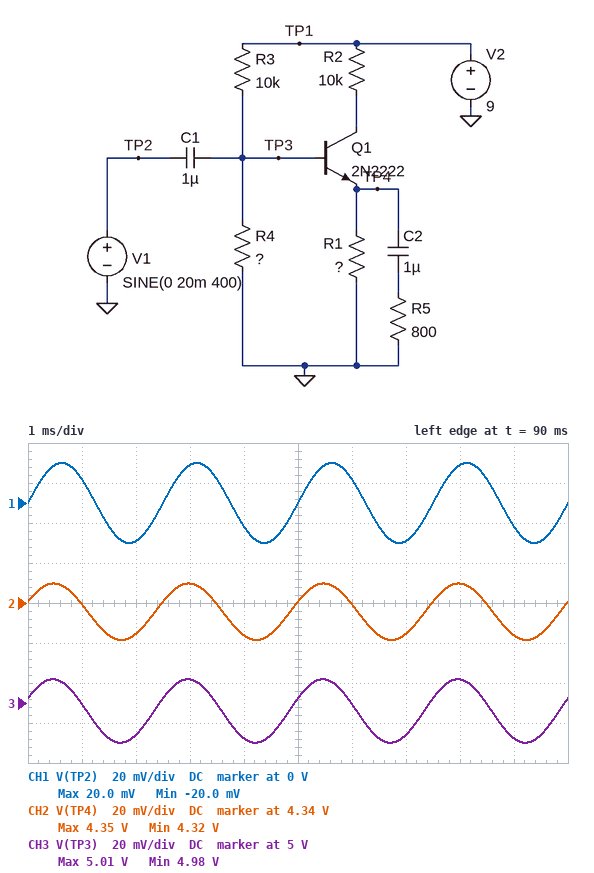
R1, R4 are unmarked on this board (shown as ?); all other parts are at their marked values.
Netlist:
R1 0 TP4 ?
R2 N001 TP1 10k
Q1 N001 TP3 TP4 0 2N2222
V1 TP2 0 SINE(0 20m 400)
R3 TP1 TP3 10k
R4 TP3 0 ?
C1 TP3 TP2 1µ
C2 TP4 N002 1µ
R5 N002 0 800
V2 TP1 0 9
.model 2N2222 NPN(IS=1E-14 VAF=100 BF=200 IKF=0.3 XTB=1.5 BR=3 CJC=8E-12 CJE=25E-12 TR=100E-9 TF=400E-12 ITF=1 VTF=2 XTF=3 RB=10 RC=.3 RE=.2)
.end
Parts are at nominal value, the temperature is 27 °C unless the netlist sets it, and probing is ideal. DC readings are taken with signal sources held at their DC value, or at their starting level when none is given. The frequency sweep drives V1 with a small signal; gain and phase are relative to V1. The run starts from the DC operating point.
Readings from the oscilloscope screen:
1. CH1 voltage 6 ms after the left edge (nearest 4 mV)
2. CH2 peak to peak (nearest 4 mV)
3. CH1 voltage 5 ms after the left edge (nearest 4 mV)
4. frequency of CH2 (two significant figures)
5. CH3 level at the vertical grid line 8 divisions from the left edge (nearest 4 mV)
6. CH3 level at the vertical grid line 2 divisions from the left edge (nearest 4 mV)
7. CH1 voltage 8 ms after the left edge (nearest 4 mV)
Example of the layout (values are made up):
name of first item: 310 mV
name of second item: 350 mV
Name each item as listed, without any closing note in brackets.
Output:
CH1 voltage 6 ms after the left edge: 12 mV
CH2 peak to peak: 28 mV
CH1 voltage 5 ms after the left edge: 0 V
frequency of CH2: 400 Hz
CH3 level at the vertical grid line 8 divisions from the left edge: 5.012 V
CH3 level at the vertical grid line 2 divisions from the left edge: 4.984 V
CH1 voltage 8 ms after the left edge: 20 mV
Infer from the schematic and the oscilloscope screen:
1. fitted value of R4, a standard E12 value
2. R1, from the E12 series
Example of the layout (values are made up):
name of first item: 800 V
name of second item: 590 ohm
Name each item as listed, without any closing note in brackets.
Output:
fitted value of R4, a standard E12 value: 22 kΩ
R1, from the E12 series: 6.8 kΩ
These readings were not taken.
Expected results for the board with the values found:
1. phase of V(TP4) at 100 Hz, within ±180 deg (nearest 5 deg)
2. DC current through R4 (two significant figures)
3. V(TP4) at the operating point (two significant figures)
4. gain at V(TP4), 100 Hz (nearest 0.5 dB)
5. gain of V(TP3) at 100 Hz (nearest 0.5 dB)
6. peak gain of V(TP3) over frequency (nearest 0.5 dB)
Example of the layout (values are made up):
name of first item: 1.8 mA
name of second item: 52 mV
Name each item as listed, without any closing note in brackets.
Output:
phase of V(TP4) at 100 Hz, within ±180 deg: 30 deg
DC current through R4: 230 µA
V(TP4) at the operating point: 4.3 V
gain at V(TP4), 100 Hz: -6.5 dB
gain of V(TP3) at 100 Hz: -6.0 dB
peak gain of V(TP3) over frequency: 0 dB
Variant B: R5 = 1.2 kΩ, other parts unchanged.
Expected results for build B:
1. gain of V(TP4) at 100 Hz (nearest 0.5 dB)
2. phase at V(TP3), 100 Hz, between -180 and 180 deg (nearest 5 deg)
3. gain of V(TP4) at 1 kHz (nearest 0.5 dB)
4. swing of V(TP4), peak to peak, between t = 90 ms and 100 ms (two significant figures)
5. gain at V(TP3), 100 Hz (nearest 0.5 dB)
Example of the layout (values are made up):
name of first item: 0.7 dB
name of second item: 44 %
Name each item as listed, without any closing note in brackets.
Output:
gain of V(TP4) at 100 Hz: -6.0 dB
phase at V(TP3), 100 Hz, between -180 and 180 deg: 35 deg
gain of V(TP4) at 1 kHz: -1.0 dB
swing of V(TP4), peak to peak, between t = 90 ms and 100 ms: 31 mV
gain at V(TP3), 100 Hz: -5.5 dB
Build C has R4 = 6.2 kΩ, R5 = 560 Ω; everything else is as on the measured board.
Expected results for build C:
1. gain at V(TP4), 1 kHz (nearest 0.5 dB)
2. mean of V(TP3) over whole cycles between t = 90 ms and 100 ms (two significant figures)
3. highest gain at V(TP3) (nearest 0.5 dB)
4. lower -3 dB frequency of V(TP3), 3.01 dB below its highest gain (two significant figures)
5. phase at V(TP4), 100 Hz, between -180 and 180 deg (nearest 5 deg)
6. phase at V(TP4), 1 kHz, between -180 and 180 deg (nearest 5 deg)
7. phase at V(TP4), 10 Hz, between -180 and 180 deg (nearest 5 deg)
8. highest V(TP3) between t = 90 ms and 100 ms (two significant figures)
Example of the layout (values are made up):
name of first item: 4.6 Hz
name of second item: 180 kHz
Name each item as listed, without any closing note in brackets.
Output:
gain at V(TP4), 1 kHz: -1.0 dB
mean of V(TP3) over whole cycles between t = 90 ms and 100 ms: 3.4 V
highest gain at V(TP3): 0 dB
lower -3 dB frequency of V(TP3), 3.01 dB below its highest gain: 42 Hz
phase at V(TP4), 100 Hz, between -180 and 180 deg: 20 deg
phase at V(TP4), 1 kHz, between -180 and 180 deg: 0 deg
phase at V(TP4), 10 Hz, between -180 and 180 deg: 75 deg
highest V(TP3) between t = 90 ms and 100 ms: 3.5 V
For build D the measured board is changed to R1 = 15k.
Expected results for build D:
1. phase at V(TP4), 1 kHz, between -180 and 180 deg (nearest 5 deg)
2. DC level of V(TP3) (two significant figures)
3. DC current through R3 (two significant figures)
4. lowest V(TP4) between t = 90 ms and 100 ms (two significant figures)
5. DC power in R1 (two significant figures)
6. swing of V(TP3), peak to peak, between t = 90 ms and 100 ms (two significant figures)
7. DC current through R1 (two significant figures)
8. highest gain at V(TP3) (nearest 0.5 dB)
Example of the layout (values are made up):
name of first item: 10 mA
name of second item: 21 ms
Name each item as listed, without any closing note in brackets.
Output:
phase at V(TP4), 1 kHz, between -180 and 180 deg: 5 deg
DC level of V(TP3): 6.1 V
DC current through R3: 290 µA
lowest V(TP4) between t = 90 ms and 100 ms: 5.4 V
DC power in R1: 2.0 mW
swing of V(TP3), peak to peak, between t = 90 ms and 100 ms: 35 mV
DC current through R1: 360 µA
highest gain at V(TP3): 0 dB
